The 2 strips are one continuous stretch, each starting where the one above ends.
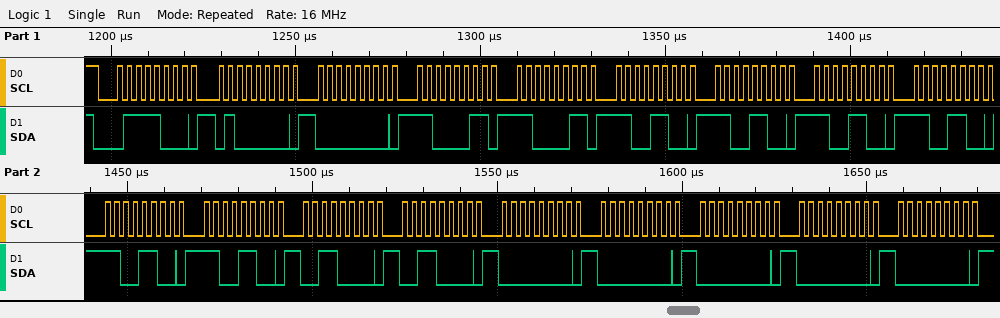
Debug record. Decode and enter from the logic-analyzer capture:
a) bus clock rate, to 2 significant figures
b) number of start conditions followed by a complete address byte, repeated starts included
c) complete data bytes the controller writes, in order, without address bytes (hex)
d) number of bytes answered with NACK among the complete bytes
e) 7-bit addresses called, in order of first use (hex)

400 kHz
1
40 00 C3 C3 CC CC CC CC CC CC 30 30 00 00 00 00 00
0
0x3C
